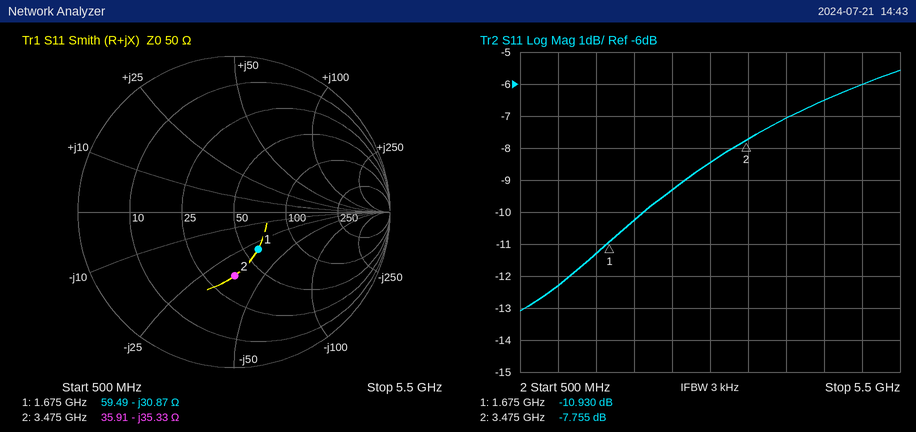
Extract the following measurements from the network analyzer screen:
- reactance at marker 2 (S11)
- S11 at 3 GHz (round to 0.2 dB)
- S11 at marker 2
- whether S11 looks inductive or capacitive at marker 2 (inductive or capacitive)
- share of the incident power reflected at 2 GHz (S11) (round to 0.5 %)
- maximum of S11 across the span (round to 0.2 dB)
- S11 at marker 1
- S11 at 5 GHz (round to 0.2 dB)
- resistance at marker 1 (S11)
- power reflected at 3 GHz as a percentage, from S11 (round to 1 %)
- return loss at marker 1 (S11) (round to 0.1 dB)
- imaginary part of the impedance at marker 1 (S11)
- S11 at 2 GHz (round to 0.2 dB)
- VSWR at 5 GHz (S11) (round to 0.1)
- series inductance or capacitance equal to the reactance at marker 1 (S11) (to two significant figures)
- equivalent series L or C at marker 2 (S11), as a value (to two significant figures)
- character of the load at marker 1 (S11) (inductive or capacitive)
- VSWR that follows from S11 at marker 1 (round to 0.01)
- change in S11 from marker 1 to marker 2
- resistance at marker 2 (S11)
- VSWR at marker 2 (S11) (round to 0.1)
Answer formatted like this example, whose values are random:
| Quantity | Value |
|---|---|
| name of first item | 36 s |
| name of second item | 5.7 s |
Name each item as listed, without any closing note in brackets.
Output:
| Quantity | Value |
|---|---|
| reactance at marker 2 | -35.33 Ω |
| S11 at 3 GHz | -8.4 dB |
| S11 at marker 2 | -7.755 dB |
| whether S11 looks inductive or capacitive at marker 2 | capacitive |
| share of the incident power reflected at 2 GHz (S11) | 9.5 % |
| maximum of S11 across the span | -5.6 dB |
| S11 at marker 1 | -10.930 dB |
| S11 at 5 GHz | -6.0 dB |
| resistance at marker 1 | 59.49 Ω |
| power reflected at 3 GHz as a percentage, from S11 | 14 % |
| return loss at marker 1 (S11) | 10.9 dB |
| imaginary part of the impedance at marker 1 | -30.87 Ω |
| S11 at 2 GHz | -10.2 dB |
| VSWR at 5 GHz (S11) | 3.0 |
| series inductance or capacitance equal to the reactance at marker 1 (S11) | 3.1 pF |
| equivalent series L or C at marker 2 (S11), as a value | 1.3 pF |
| character of the load at marker 1 (S11) | capacitive |
| VSWR that follows from S11 at marker 1 | 1.79 |
| change in S11 from marker 1 to marker 2 | 3.175 dB |
| resistance at marker 2 | 35.91 Ω |
| VSWR at marker 2 (S11) | 2.4 |
